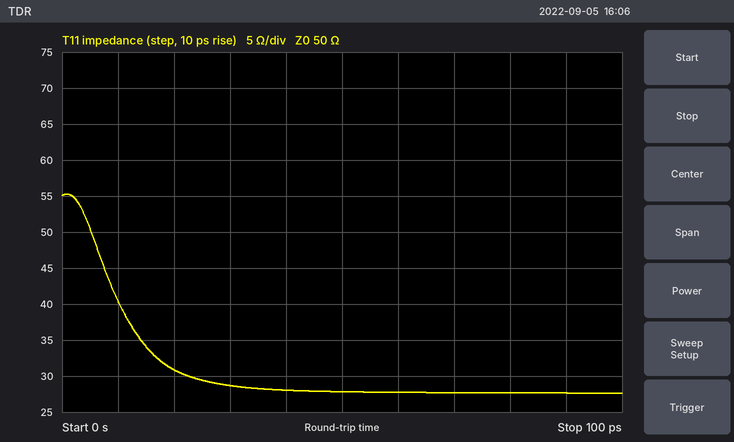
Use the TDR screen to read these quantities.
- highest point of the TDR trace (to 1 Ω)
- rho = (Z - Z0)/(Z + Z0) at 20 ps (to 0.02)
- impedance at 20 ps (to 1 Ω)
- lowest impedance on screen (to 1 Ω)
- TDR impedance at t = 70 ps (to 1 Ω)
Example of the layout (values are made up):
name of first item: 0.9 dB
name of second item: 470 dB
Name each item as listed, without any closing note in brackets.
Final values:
highest point of the TDR trace: 55 Ω
rho = (Z - Z0)/(Z + Z0) at 20 ps: -0.24
impedance at 20 ps: 31 Ω
lowest impedance on screen: 28 Ω
TDR impedance at t = 70 ps: 28 Ω
